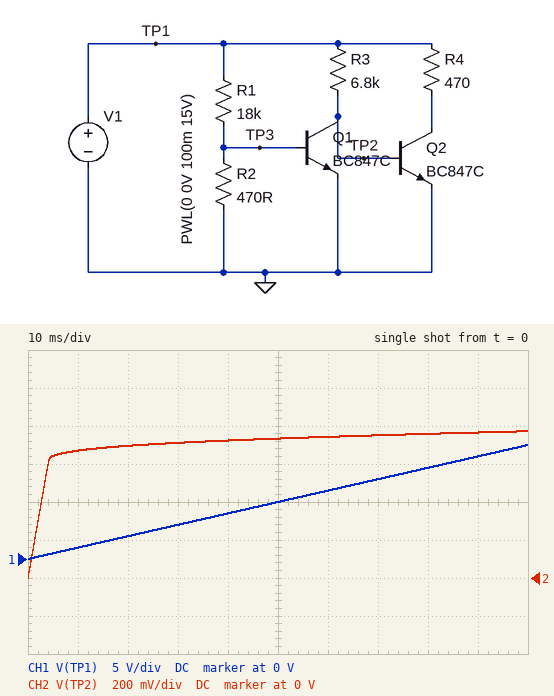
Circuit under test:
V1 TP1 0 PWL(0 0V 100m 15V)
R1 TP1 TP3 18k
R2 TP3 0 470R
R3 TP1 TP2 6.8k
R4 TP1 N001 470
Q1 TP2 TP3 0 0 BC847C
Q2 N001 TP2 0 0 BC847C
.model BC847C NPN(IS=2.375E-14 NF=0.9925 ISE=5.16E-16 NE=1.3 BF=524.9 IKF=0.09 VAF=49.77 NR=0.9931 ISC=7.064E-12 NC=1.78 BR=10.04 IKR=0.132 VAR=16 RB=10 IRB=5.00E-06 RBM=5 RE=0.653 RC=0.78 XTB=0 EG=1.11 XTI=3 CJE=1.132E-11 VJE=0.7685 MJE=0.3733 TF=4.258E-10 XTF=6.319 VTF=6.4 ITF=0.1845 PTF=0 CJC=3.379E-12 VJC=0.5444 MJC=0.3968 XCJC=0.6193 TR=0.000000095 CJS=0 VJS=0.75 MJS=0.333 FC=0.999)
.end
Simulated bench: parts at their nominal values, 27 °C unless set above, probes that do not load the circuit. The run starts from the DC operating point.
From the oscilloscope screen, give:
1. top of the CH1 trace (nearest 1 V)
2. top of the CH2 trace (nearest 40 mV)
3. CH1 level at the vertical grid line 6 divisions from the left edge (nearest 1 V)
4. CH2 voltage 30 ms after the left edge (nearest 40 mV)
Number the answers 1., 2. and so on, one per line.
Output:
1. 15 V
2. 760 mV
3. 9 V
4. 720 mV
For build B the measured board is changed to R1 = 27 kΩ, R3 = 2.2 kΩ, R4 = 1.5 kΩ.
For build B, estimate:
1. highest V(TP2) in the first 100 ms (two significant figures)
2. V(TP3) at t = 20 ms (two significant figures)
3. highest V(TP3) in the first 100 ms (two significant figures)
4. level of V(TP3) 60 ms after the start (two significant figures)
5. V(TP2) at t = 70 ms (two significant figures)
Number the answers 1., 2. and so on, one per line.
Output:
1. 790 mV
2. 51 mV
3. 260 mV
4. 150 mV
5. 760 mV
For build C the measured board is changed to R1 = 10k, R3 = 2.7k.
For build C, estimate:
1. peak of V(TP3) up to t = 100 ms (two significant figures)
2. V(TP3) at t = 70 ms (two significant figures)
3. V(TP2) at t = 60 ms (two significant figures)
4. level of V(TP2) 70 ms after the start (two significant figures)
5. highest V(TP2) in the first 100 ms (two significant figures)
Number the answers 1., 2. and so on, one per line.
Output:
1. 670 mV
2. 470 mV
3. 770 mV
4. 780 mV
5. 790 mV
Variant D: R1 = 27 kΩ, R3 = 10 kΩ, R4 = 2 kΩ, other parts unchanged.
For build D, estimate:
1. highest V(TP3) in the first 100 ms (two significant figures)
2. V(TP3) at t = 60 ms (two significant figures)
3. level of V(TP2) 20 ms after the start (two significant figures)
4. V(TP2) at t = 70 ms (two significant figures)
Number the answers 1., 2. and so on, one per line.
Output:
1. 260 mV
2. 150 mV
3. 670 mV
4. 710 mV
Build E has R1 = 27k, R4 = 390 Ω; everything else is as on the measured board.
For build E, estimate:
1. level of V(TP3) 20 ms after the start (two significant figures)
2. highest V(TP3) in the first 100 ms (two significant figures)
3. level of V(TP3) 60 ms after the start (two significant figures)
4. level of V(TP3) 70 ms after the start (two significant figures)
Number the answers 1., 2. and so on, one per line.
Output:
1. 51 mV
2. 260 mV
3. 150 mV
4. 180 mV
